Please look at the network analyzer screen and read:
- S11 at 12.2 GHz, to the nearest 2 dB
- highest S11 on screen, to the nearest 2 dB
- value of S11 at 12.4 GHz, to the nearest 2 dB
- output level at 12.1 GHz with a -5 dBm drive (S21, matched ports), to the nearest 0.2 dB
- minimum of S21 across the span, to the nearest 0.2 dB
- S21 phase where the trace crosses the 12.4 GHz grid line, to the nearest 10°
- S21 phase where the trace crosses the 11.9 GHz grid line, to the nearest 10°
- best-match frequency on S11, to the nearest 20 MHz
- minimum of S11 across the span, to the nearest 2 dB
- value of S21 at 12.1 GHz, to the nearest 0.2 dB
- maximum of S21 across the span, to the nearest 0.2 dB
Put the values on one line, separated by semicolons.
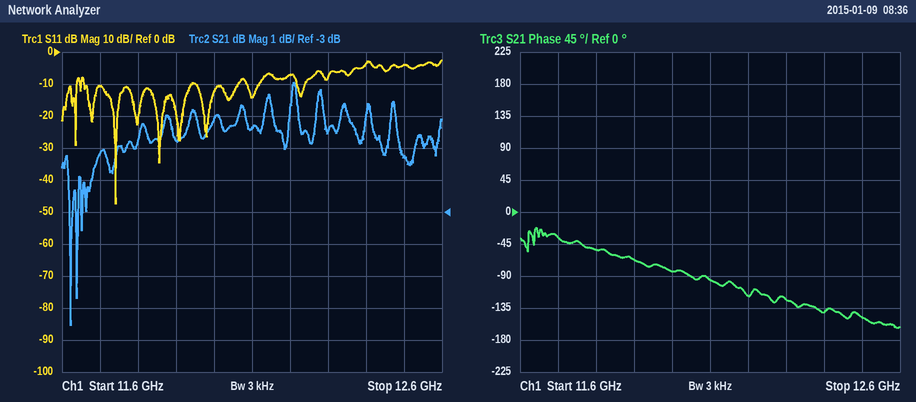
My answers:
-8 dB; -2 dB; -4 dB; -5.4 dBm; -6.6 dB; -140°; -70°; 11.74 GHz; -48 dB; -0.4 dB; 1.0 dB
